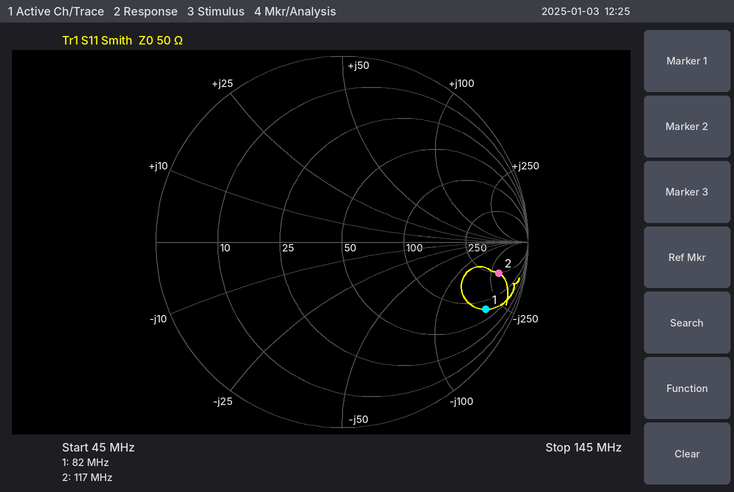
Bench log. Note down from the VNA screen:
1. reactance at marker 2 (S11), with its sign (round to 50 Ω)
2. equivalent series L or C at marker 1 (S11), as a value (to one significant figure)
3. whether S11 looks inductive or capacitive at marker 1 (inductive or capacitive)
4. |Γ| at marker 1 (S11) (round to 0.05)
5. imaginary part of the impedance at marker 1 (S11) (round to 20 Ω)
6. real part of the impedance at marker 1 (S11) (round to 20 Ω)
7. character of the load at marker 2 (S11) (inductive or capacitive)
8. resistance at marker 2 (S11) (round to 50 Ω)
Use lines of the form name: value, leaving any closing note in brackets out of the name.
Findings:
reactance at marker 2 (S11), with its sign: -300 Ω
equivalent series L or C at marker 1 (S11), as a value: 10 pF
whether S11 looks inductive or capacitive at marker 1: capacitive
|Γ| at marker 1 (S11): 0.85
imaginary part of the impedance at marker 1 (S11): -200 Ω
real part of the impedance at marker 1 (S11): 80 Ω
character of the load at marker 2 (S11): capacitive
resistance at marker 2 (S11): 250 Ω
